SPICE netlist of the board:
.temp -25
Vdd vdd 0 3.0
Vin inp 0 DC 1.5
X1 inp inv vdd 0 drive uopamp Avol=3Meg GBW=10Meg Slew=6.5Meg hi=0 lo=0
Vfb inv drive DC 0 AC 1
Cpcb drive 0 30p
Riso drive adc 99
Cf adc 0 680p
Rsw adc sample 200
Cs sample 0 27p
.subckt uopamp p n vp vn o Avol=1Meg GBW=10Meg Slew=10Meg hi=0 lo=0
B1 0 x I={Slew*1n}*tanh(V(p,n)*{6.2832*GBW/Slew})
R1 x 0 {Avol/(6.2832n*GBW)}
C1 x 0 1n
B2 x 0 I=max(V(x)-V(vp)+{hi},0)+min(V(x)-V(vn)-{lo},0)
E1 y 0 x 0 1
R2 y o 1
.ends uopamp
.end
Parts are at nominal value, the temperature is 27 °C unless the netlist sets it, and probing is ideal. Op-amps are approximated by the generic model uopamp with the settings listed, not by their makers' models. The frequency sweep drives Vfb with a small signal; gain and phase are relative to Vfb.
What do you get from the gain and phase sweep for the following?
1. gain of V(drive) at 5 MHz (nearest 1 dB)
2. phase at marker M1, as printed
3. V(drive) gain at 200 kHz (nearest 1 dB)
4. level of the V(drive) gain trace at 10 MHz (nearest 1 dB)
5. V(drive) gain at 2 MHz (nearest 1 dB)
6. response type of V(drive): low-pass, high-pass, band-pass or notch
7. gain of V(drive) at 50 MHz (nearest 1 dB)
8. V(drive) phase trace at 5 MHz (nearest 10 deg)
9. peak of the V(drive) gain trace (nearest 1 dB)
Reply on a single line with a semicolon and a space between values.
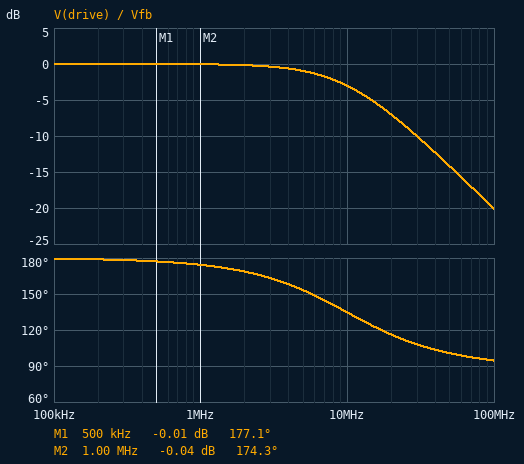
-1 dB; 177.1 deg; 0 dB; -3 dB; 0 dB; low-pass; -14 dB; 150 deg; 0 dB
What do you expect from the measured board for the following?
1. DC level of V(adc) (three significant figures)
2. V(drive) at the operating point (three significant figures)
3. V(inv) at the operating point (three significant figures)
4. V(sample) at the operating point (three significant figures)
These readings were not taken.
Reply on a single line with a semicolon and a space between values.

1.50 V; 1.50 V; 1.50 V; 1.50 V
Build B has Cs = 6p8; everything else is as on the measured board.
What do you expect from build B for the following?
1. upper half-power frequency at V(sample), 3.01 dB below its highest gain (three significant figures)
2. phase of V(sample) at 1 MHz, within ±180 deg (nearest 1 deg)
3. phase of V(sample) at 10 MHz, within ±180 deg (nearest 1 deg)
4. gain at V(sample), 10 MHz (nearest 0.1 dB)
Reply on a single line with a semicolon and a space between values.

2.23 MHz; 151 deg; 53 deg; -15.9 dB
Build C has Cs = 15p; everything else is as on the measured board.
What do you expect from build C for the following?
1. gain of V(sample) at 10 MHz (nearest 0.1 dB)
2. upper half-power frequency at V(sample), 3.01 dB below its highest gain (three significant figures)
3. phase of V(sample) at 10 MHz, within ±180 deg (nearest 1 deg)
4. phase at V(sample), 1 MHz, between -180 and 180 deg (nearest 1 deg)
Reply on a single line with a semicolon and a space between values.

-16.1 dB; 2.20 MHz; 47 deg; 150 deg
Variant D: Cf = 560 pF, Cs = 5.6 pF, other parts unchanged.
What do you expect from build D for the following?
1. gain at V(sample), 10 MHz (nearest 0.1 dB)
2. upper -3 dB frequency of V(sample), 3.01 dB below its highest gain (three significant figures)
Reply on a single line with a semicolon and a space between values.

-14.3 dB; 2.65 MHz
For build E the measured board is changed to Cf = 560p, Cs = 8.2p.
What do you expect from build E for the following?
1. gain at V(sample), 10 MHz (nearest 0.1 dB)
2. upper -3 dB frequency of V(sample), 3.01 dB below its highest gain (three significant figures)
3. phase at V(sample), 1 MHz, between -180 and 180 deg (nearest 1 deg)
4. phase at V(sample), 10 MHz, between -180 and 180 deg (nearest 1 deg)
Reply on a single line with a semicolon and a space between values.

-14.4 dB; 2.64 MHz; 154 deg; 55 deg
